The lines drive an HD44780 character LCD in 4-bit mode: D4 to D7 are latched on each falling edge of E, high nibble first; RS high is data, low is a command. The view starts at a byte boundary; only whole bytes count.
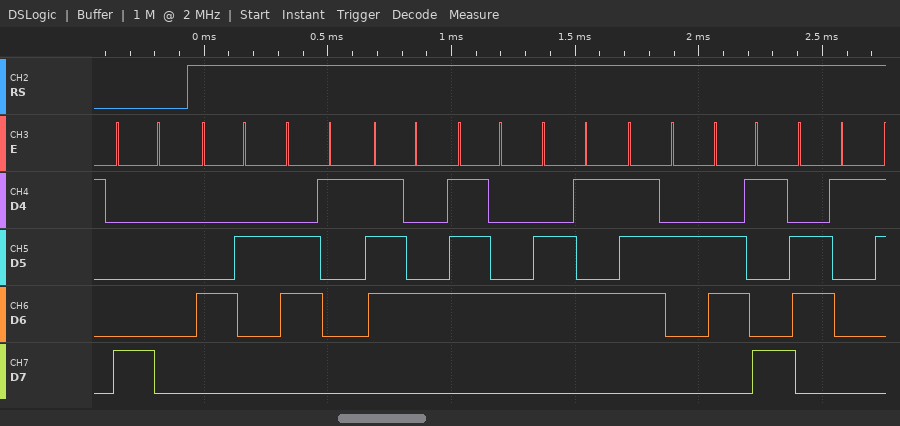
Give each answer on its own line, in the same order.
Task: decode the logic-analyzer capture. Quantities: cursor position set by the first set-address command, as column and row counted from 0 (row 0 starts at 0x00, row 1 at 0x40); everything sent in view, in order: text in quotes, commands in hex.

column 0, row 0
0x80 "Batteria"
